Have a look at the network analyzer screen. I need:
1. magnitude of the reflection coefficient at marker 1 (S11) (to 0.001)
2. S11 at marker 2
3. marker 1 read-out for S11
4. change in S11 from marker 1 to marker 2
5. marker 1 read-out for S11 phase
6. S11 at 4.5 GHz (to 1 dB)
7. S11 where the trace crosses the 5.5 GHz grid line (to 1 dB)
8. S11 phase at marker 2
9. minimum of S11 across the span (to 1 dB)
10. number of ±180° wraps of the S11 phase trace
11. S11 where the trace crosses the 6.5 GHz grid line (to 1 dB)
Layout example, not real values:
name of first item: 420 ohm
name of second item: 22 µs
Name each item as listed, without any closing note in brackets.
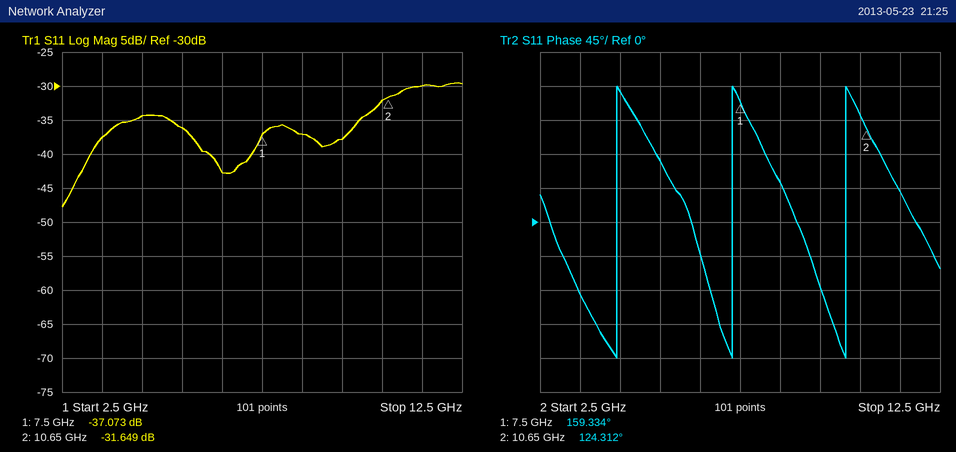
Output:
magnitude of the reflection coefficient at marker 1 (S11): 0.014
S11 at marker 2: -31.649 dB
marker 1 read-out for S11: -37.073 dB
change in S11 from marker 1 to marker 2: 5.424 dB
marker 1 read-out for S11 phase: 159.334°
S11 at 4.5 GHz: -34 dB
S11 where the trace crosses the 5.5 GHz grid line: -36 dB
S11 phase at marker 2: 124.312°
minimum of S11 across the span: -48 dB
number of ±180° wraps of the S11 phase trace: 3
S11 where the trace crosses the 6.5 GHz grid line: -43 dB
